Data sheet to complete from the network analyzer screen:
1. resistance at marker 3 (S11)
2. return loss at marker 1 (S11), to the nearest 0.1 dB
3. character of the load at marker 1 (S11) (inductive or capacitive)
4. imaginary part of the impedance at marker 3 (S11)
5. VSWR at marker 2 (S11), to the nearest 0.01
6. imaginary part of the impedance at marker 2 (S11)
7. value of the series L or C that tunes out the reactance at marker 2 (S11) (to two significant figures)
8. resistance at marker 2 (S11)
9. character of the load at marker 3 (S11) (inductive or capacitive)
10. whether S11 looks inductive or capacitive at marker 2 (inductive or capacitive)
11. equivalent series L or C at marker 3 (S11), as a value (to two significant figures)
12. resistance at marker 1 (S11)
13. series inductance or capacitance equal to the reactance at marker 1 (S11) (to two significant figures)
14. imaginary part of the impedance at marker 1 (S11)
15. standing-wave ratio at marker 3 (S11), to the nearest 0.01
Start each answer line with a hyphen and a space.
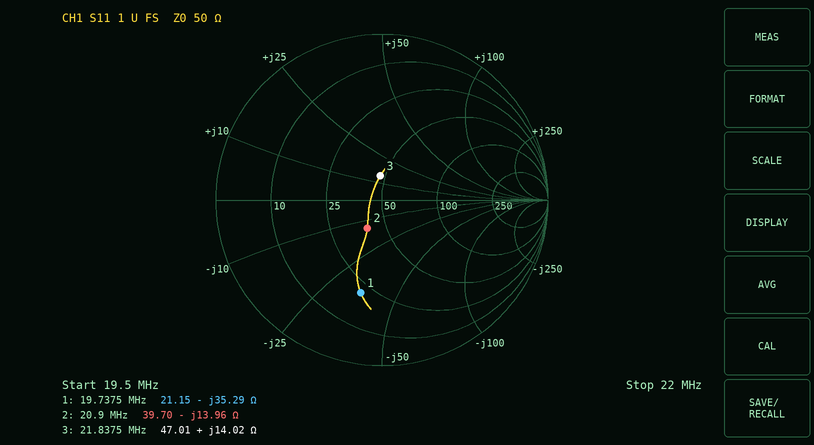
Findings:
- 47.01 Ω
- 4.8 dB
- capacitive
- +14.02 Ω
- 1.47
- -13.96 Ω
- 110 nH
- 39.70 Ω
- inductive
- capacitive
- 100 nH
- 21.15 Ω
- 230 pF
- -35.29 Ω
- 1.34
